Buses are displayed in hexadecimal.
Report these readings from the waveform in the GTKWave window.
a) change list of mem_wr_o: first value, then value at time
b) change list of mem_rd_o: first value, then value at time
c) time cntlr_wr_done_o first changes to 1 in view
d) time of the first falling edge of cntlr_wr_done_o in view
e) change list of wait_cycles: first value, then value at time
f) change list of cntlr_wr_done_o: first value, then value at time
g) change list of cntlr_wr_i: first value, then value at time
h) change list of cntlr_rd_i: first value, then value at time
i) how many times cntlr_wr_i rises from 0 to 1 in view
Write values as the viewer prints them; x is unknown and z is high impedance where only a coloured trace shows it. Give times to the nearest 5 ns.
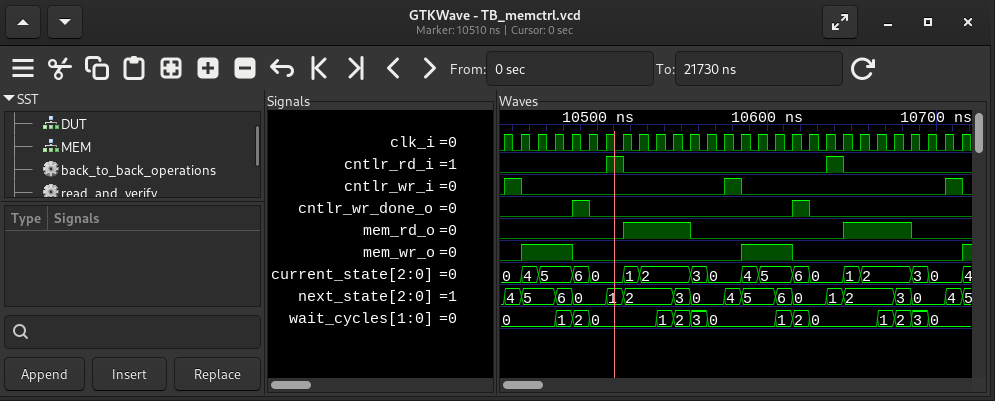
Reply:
0, 1 at 10455 ns, 0 at 10485 ns, 1 at 10585 ns, 0 at 10615 ns, 1 at 10715 ns
0, 1 at 10515 ns, 0 at 10555 ns, 1 at 10645 ns, 0 at 10685 ns
10485 ns
10495 ns
0, 1 at 10475 ns, 2 at 10485 ns, 0 at 10495 ns, 1 at 10535 ns, 2 at 10545 ns, 3 at 10555 ns, 0 at 10565 ns, 1 at 10605 ns, 2 at 10615 ns, 0 at 10625 ns, 1 at 10665 ns, 2 at 10675 ns, 3 at 10685 ns, 0 at 10695 ns
0, 1 at 10485 ns, 0 at 10495 ns, 1 at 10615 ns, 0 at 10625 ns
0, 1 at 10445 ns, 0 at 10455 ns, 1 at 10575 ns, 0 at 10585 ns, 1 at 10705 ns, 0 at 10715 ns
0, 1 at 10505 ns, 0 at 10515 ns, 1 at 10635 ns, 0 at 10645 ns
3
